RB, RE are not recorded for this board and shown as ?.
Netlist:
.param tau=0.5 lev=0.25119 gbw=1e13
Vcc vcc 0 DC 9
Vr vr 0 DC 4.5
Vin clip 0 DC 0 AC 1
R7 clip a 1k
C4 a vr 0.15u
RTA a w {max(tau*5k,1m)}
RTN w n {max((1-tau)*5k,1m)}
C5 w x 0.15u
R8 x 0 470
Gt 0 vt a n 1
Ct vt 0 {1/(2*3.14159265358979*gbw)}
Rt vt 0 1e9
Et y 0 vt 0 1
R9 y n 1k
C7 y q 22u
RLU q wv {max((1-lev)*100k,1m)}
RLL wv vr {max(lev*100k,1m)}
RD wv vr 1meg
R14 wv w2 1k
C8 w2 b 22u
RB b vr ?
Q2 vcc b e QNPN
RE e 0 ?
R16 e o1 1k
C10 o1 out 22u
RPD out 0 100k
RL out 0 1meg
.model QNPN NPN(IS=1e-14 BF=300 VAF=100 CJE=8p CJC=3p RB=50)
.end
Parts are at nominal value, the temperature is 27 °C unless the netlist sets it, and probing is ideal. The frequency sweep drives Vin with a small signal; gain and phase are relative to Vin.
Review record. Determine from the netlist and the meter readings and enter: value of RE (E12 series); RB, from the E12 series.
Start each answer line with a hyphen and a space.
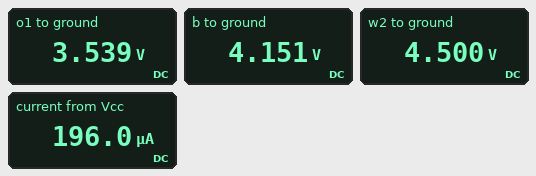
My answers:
- 18 kΩ
- 560 kΩ
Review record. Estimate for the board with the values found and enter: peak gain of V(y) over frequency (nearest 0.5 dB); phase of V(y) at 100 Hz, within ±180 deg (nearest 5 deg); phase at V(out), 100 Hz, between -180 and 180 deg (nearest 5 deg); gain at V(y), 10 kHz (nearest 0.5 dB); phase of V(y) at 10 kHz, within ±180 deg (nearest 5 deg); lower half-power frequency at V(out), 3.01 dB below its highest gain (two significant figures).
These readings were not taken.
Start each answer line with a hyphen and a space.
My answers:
- 0 dB
- -5 deg
- -5 deg
- -17.5 dB
- -80 deg
- 120 mHz
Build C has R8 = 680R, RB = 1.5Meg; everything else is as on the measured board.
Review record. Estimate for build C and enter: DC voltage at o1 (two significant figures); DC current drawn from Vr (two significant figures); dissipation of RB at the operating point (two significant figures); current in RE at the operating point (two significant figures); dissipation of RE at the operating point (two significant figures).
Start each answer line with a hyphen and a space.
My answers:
- 3.1 V
- 540 nA
- 440 nW
- 170 µA
- 530 µW
